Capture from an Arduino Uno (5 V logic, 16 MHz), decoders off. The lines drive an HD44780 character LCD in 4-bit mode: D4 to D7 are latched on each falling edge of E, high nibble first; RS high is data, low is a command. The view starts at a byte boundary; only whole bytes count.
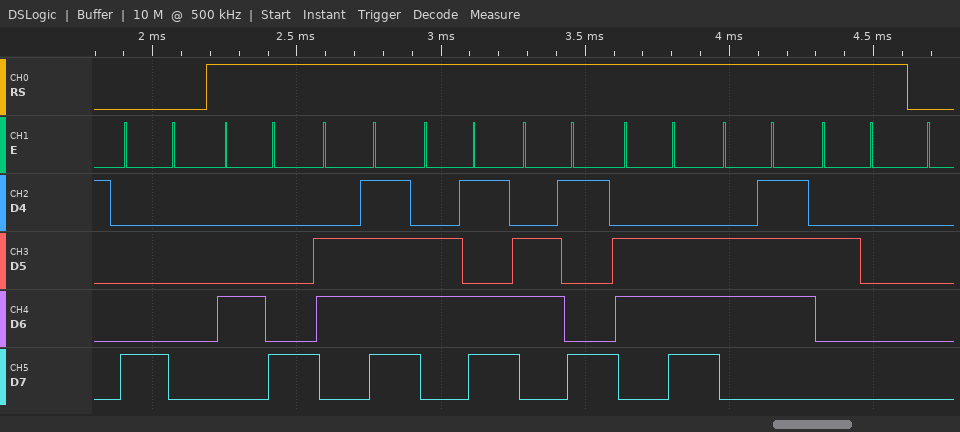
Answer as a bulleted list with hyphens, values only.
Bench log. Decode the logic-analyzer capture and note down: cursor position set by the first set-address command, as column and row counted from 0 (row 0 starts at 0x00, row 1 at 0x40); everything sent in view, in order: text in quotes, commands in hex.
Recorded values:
- column 0, row 0
- 0x80 "Homing "
